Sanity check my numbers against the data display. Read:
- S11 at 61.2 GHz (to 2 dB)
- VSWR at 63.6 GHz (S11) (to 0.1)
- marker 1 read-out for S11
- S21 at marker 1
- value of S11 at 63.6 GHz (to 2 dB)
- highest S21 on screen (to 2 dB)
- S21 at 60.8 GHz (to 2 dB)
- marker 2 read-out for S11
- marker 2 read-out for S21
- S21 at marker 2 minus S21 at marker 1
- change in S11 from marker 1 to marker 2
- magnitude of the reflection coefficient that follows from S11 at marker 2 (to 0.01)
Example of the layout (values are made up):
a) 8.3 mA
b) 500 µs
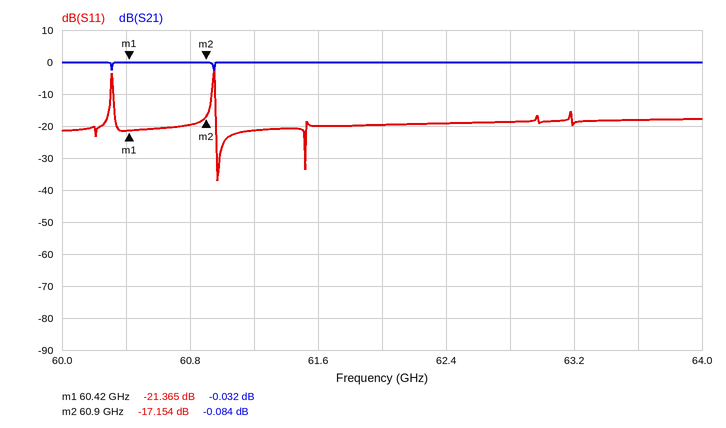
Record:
a) -22 dB
b) 1.3
c) -21.365 dB
d) -0.032 dB
e) -18 dB
f) 0 dB
g) 0 dB
h) -17.154 dB
i) -0.084 dB
j) -0.052 dB
k) 4.211 dB
l) 0.14
